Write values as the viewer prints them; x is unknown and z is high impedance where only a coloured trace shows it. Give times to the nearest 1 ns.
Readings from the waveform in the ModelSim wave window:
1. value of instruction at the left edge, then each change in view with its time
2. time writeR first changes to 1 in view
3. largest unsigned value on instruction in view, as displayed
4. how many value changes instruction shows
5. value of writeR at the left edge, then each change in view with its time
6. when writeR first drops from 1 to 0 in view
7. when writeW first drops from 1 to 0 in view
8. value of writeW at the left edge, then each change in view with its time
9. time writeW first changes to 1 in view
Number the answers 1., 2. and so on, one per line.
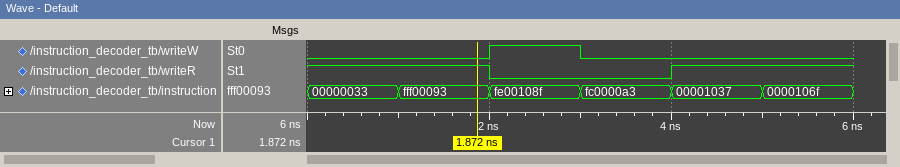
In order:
1. 00000033, fff00093 at 1 ns, fe00108f at 2 ns, fc0000a3 at 3 ns, 00001037 at 4 ns, 0000106f at 5 ns
2. 4 ns
3. fff00093
4. 5
5. 1, 0 at 2 ns, 1 at 4 ns
6. 2 ns
7. 3 ns
8. 0, 1 at 2 ns, 0 at 3 ns
9. 2 ns
